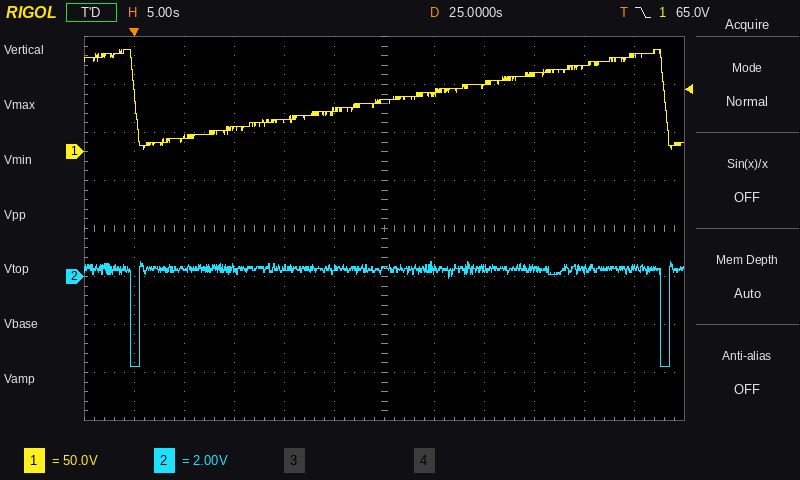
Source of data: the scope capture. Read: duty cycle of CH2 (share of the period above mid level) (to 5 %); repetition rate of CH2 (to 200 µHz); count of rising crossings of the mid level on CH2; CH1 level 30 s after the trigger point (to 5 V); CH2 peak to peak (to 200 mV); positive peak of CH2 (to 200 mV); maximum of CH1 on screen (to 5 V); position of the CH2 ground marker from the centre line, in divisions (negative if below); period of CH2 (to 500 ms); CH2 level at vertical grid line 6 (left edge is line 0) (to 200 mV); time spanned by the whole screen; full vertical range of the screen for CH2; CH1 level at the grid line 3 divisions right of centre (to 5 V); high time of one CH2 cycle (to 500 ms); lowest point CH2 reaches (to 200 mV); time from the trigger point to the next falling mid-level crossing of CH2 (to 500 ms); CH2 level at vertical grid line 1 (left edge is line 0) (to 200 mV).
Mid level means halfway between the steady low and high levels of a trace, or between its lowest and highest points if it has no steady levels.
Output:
100 %
18.8 mHz
2
60 V
4.4 V
600 mV
105 V
-1.0 div
53.0 s
400 mV
60 s
16 V
80 V
52.0 s
-3.8 V
52.5 s
-3.8 V
